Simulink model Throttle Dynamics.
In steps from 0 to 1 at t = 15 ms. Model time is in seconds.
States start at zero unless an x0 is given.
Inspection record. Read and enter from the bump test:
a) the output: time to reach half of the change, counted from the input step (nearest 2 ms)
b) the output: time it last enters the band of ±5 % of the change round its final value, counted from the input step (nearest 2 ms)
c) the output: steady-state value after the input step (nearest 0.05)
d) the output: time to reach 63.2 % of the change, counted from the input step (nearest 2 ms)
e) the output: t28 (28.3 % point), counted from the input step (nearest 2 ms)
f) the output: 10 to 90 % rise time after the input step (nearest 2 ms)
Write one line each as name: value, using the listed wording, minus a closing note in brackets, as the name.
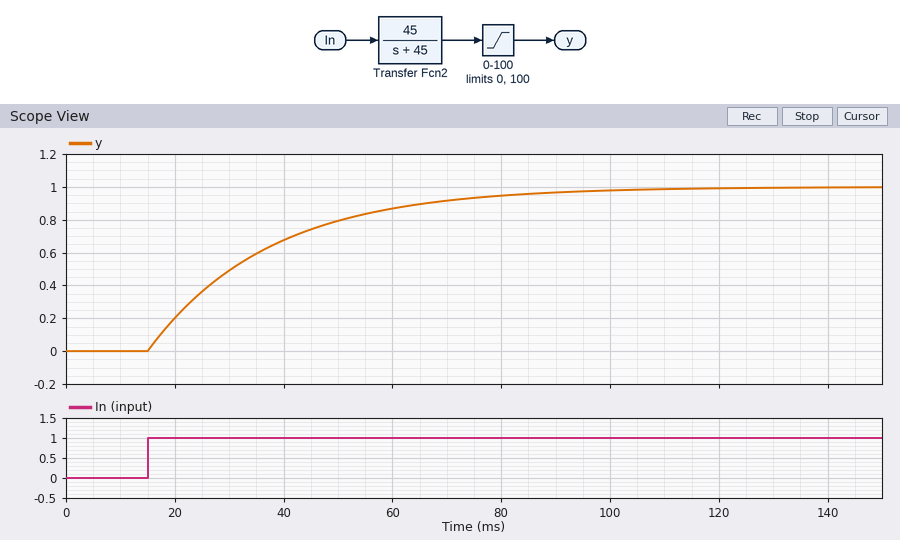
the output: time to reach half of the change, counted from the input step: 16 ms
the output: time it last enters the band of ±5 % of the change round its final value, counted from the input step: 66 ms
the output: steady-state value after the input step: 1.00
the output: time to reach 63.2 % of the change, counted from the input step: 22 ms
the output: t28 (28.3 % point), counted from the input step: 8 ms
the output: 10 to 90 % rise time after the input step: 48 ms
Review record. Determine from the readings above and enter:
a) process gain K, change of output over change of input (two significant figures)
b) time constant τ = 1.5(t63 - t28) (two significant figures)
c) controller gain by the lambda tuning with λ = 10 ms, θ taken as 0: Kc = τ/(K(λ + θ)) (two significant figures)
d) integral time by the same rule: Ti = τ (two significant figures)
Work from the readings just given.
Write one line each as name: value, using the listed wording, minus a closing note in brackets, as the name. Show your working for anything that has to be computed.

process gain K, change of output over change of input: (1 - 0) / 1 = 1.0
time constant τ = 1.5(t63 - t28): 1.5 × (22 - 8) = 21 ms
controller gain by the lambda tuning with λ = 10 ms, θ taken as 0: Kc = τ/(K(λ + θ)): 21 / (1 × (10 + 0)) = 2.1
integral time by the same rule: Ti = τ: 21 ms
